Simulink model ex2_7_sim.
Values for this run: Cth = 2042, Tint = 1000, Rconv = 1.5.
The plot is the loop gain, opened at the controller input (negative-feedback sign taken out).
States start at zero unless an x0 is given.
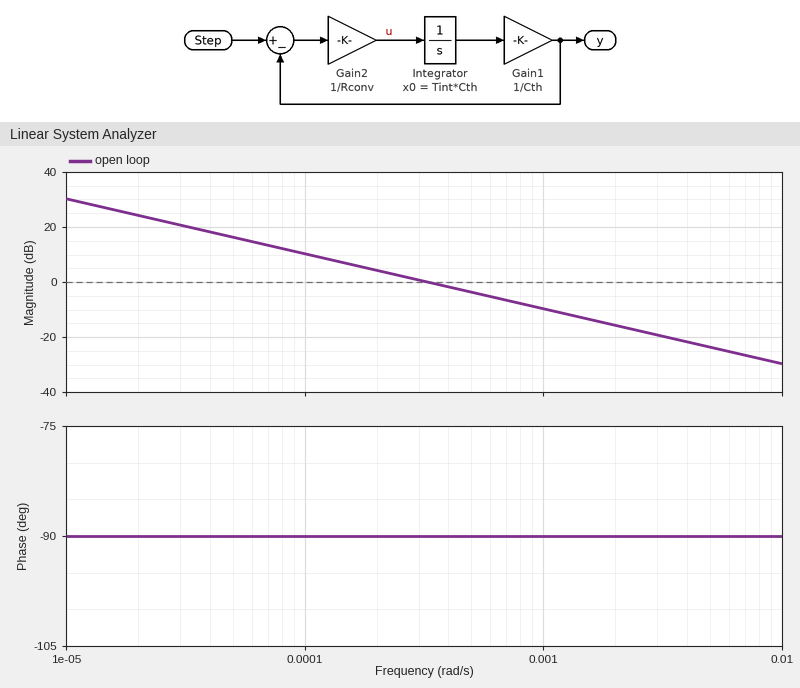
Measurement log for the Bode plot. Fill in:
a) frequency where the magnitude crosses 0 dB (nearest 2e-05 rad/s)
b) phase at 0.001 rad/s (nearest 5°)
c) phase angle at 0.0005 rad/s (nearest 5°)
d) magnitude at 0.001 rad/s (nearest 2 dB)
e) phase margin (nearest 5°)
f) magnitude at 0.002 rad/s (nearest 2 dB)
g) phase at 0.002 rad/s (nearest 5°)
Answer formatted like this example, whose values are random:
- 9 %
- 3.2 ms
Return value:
- 0.00032 rad/s
- -90°
- -90°
- -10 dB
- 90°
- -16 dB
- -90°
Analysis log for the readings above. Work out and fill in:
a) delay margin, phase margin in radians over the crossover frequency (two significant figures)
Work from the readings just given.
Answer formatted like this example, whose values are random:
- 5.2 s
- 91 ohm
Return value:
- 4900 s
